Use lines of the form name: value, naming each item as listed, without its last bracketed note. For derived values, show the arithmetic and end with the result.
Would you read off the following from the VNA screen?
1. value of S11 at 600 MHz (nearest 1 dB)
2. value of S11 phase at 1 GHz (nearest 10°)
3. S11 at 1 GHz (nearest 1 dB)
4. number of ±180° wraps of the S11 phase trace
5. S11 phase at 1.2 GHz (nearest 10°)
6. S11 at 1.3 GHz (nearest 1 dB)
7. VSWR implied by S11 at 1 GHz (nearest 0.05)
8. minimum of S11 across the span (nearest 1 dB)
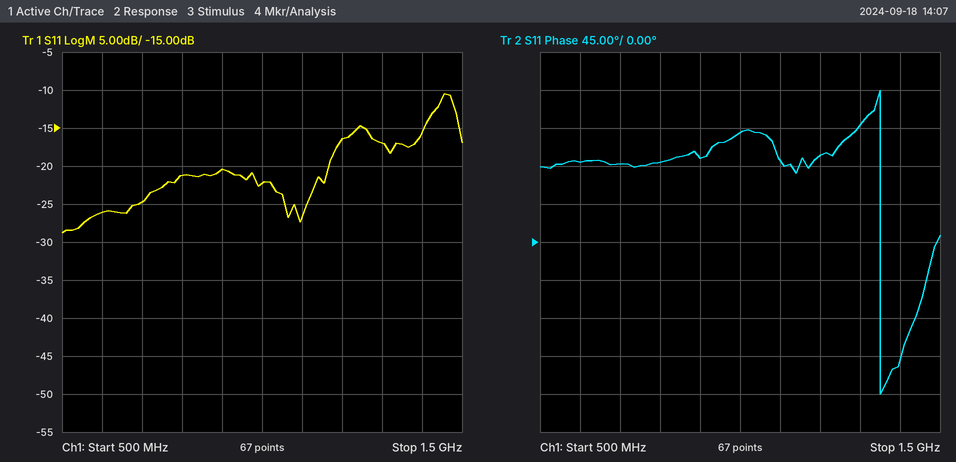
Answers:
value of S11 at 600 MHz: -26 dB
value of S11 phase at 1 GHz: 130°
S11 at 1 GHz: -22 dB
number of ±180° wraps of the S11 phase trace: 1
S11 phase at 1.2 GHz: 100°
S11 at 1.3 GHz: -17 dB
VSWR implied by S11 at 1 GHz: |Γ| = 10^(-22/20) = 0.0794; VSWR = (1 + 0.0794)/(1 − 0.0794) ≈ 1.17, so 1.15 to the nearest 0.05
minimum of S11 across the span: -29 dB
